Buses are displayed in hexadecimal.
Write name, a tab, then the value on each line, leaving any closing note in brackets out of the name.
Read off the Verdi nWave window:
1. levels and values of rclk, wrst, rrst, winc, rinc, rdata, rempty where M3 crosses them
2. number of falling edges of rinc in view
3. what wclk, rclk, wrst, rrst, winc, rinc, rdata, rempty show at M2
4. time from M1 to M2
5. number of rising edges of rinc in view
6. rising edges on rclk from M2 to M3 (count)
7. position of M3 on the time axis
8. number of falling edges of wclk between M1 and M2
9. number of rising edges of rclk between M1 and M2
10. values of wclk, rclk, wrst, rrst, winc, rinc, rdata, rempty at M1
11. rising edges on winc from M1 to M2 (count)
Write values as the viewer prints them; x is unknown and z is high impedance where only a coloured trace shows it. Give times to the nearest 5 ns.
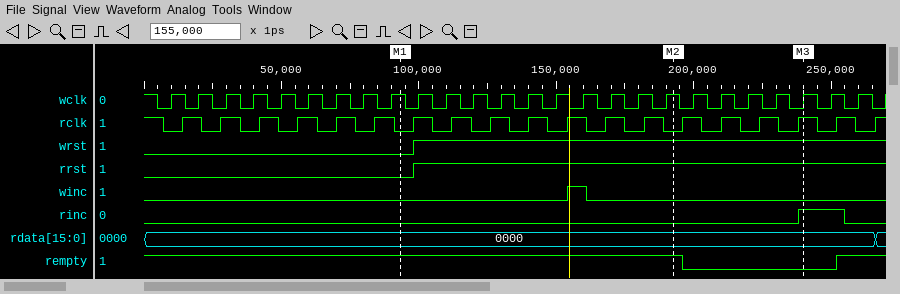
levels and values of rclk, wrst, rrst, winc, rinc, rdata, rempty where M3 crosses them	rclk=1, wrst=1, rrst=1, winc=0, rinc=1, rdata=0000, rempty=0
number of falling edges of rinc in view	1
what wclk, rclk, wrst, rrst, winc, rinc, rdata, rempty show at M2	wclk=1, rclk=0, wrst=1, rrst=1, winc=0, rinc=0, rdata=0000, rempty=1
time from M1 to M2	100 ns
number of rising edges of rinc in view	1
rising edges on rclk from M2 to M3	4
position of M3 on the time axis	240 ns
number of falling edges of wclk between M1 and M2	10
number of rising edges of rclk between M1 and M2	7
values of wclk, rclk, wrst, rrst, winc, rinc, rdata, rempty at M1	wclk=1, rclk=0, wrst=0, rrst=0, winc=0, rinc=0, rdata=0000, rempty=1
rising edges on winc from M1 to M2	1
